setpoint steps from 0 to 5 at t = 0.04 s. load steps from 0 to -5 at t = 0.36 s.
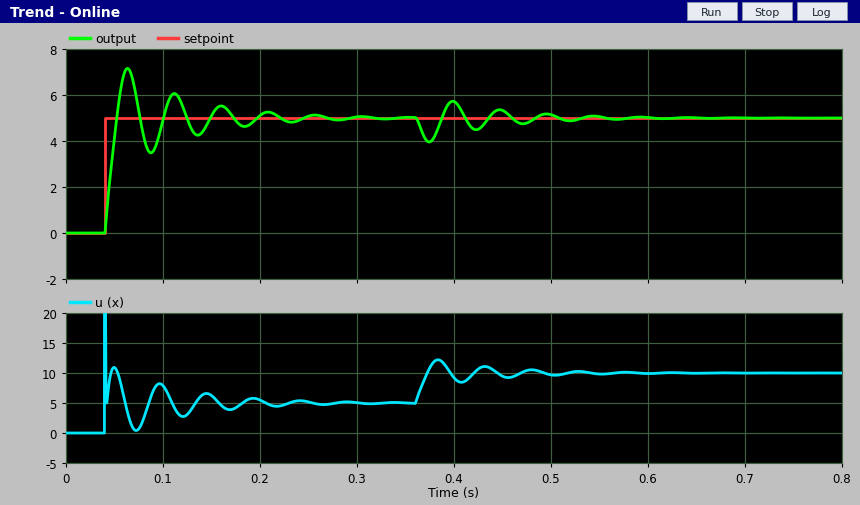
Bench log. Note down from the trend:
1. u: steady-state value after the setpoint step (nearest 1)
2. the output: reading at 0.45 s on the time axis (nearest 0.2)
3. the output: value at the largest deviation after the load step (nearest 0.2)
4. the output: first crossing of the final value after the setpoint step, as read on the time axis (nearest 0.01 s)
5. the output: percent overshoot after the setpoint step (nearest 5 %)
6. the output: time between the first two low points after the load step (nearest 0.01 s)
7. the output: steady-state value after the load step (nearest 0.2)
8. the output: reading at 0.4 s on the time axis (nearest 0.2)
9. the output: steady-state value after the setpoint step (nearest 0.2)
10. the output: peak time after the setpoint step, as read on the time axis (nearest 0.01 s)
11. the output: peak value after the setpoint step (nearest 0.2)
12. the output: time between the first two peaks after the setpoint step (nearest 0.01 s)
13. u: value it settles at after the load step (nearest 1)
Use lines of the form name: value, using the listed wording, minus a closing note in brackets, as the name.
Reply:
u: steady-state value after the setpoint step: 5
the output: reading at 0.45 s on the time axis: 5.4
the output: value at the largest deviation after the load step: 4.0
the output: first crossing of the final value after the setpoint step, as read on the time axis: 0.05 s
the output: percent overshoot after the setpoint step: 45 %
the output: time between the first two low points after the load step: 0.05 s
the output: steady-state value after the load step: 5.0
the output: reading at 0.4 s on the time axis: 5.8
the output: steady-state value after the setpoint step: 5.0
the output: peak time after the setpoint step, as read on the time axis: 0.06 s
the output: peak value after the setpoint step: 7.2
the output: time between the first two peaks after the setpoint step: 0.05 s
u: value it settles at after the load step: 10
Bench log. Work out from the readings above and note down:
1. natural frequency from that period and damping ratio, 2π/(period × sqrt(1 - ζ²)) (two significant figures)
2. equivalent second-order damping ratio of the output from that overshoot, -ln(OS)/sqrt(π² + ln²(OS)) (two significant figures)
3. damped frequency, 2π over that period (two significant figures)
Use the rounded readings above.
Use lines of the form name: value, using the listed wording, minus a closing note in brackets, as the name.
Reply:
natural frequency from that period and damping ratio, 2π/(period × sqrt(1 - ζ²)): 130 rad/s
equivalent second-order damping ratio of the output from that overshoot, -ln(OS)/sqrt(π² + ln²(OS)): 0.25
damped frequency, 2π over that period: 130 rad/s
